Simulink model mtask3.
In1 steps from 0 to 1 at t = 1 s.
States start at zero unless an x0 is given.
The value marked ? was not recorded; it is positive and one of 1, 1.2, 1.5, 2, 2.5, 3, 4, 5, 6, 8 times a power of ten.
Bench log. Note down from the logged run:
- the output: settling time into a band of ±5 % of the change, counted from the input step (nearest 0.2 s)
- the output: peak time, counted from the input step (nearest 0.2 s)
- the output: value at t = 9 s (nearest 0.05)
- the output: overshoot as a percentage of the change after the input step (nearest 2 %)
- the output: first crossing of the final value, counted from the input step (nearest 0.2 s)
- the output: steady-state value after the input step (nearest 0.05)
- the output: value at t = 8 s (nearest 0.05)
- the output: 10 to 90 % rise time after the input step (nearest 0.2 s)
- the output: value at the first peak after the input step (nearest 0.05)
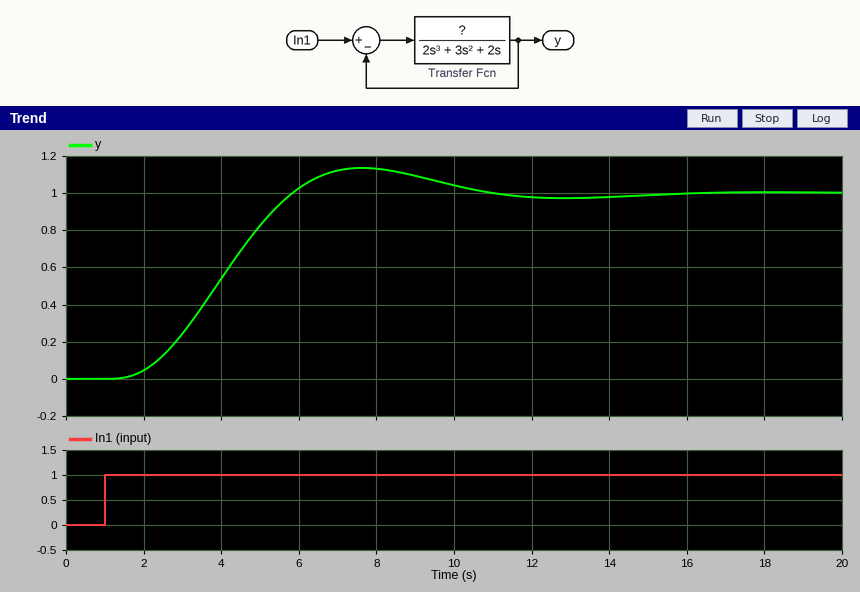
8.8 s
6.6 s
1.10
14 %
4.8 s
1.00
1.15
3.0 s
1.15
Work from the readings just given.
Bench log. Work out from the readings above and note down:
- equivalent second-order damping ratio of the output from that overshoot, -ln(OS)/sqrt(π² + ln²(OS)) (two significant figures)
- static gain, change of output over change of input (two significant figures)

0.53
1.0
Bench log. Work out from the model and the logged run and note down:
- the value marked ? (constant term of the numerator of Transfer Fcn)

0.8
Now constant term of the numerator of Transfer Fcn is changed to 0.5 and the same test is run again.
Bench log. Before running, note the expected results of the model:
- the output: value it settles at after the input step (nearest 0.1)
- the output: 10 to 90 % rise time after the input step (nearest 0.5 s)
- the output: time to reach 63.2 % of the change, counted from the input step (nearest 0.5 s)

1.0
5.0 s
4.5 s
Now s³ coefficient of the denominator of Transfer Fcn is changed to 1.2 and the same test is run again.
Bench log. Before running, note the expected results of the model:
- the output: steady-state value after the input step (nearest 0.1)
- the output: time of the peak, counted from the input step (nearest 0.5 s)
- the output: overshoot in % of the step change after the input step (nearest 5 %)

1.0
7.0 s
10 %
